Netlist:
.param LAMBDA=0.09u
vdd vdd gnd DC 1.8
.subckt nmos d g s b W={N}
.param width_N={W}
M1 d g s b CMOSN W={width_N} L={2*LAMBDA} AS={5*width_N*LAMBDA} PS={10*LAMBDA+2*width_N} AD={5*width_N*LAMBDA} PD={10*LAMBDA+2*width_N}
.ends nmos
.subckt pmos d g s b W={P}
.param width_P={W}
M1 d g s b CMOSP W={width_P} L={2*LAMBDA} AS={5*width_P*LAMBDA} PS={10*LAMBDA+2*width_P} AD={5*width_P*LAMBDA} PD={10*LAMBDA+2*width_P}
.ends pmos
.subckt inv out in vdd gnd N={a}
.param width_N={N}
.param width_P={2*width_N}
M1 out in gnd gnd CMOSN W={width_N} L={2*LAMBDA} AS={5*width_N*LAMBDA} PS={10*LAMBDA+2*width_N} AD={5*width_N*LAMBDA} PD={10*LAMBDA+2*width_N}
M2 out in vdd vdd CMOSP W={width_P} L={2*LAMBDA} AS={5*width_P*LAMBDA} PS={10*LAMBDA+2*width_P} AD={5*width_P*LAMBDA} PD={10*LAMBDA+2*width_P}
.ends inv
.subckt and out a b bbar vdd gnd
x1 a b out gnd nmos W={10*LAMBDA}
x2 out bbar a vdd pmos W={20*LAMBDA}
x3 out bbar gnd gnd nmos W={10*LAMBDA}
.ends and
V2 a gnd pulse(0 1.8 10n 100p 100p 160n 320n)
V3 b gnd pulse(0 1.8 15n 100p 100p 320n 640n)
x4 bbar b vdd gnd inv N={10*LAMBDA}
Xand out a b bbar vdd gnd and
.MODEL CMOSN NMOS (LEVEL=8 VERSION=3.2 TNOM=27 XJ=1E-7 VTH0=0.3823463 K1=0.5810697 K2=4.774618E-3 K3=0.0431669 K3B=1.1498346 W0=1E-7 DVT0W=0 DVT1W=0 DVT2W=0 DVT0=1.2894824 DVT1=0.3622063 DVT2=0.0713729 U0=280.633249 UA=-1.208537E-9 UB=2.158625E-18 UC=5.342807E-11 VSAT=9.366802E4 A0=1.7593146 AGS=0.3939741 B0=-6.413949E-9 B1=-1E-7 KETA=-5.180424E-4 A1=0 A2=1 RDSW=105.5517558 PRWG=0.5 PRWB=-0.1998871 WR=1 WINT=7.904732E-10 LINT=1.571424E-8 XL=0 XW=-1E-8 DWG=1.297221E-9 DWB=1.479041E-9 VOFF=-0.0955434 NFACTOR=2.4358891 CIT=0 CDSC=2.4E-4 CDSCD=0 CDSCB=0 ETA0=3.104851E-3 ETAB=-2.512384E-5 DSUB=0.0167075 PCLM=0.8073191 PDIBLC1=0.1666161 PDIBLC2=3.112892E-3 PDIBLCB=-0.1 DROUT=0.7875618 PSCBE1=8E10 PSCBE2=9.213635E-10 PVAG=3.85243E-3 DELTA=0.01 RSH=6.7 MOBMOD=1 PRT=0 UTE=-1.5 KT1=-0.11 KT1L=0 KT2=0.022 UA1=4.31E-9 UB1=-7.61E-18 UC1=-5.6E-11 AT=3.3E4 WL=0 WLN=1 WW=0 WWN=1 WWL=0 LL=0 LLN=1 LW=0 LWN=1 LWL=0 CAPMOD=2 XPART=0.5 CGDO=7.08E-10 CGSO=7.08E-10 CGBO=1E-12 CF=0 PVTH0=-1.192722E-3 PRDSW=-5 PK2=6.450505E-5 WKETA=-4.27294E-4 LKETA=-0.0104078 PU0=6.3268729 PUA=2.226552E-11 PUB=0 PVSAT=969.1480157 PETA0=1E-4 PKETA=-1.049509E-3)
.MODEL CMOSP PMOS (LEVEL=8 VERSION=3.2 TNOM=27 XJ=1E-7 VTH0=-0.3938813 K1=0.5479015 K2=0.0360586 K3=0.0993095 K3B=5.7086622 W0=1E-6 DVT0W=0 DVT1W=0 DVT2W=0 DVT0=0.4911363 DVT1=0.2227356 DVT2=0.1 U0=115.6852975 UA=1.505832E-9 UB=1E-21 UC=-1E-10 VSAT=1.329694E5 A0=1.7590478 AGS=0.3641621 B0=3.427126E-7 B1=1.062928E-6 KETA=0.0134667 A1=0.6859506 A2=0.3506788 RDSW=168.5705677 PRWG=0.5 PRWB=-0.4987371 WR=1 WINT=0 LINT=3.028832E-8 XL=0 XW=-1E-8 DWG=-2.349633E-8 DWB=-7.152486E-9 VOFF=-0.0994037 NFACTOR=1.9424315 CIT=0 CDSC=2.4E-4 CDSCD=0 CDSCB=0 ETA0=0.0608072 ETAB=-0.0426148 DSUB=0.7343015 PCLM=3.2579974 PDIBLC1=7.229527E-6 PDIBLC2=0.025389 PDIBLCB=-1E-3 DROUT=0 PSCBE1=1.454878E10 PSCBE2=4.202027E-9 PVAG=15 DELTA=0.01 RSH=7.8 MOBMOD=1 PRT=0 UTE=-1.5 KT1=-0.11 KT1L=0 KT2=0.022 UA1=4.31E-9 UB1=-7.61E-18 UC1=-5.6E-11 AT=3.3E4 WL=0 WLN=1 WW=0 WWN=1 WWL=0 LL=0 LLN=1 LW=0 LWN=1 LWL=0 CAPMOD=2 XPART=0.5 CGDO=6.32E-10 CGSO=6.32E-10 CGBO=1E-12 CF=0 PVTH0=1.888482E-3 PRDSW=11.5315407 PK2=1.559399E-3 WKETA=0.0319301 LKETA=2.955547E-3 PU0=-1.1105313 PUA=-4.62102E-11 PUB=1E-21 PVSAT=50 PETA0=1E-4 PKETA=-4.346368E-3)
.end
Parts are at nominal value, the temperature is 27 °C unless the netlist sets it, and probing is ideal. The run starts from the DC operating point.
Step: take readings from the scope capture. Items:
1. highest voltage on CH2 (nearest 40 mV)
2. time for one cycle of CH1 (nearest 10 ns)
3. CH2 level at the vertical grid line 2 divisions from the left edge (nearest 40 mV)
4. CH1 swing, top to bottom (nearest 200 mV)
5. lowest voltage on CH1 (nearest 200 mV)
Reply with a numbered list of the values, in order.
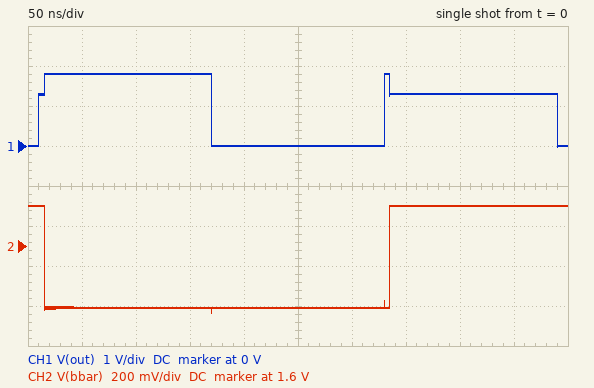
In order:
1. 1.80 V
2. 320 ns
3. 1.28 V
4. 1.8 V
5. 0 V
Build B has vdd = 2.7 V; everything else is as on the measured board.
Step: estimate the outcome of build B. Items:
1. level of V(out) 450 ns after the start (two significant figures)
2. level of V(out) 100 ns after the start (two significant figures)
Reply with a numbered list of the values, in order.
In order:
1. 22 mV
2. 480 mV
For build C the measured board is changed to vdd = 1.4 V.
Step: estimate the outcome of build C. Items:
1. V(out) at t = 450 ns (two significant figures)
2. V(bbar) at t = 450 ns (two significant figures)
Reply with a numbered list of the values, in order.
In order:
1. 1.8 V
2. 1.4 V
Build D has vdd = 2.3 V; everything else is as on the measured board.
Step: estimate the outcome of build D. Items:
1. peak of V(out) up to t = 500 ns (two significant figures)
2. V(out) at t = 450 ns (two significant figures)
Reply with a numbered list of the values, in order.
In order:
1. 500 mV
2. 22 mV
